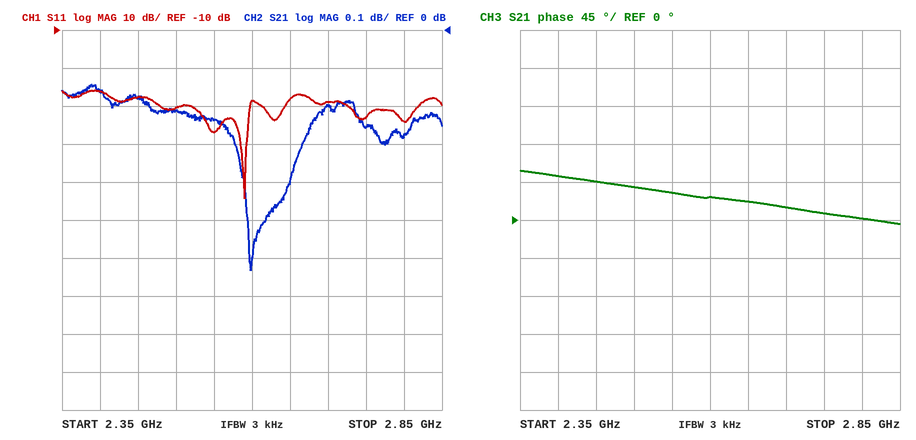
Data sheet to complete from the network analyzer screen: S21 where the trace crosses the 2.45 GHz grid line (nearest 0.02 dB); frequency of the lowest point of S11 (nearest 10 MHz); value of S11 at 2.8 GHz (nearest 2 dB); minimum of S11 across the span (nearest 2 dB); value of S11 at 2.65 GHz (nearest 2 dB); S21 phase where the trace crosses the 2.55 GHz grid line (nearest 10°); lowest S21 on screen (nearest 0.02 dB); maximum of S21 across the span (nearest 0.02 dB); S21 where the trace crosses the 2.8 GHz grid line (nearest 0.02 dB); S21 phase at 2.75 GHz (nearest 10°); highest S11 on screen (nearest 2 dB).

-0.18 dB
2.59 GHz
-34 dB
-54 dB
-28 dB
30°
-0.64 dB
-0.14 dB
-0.28 dB
10°
-26 dB
